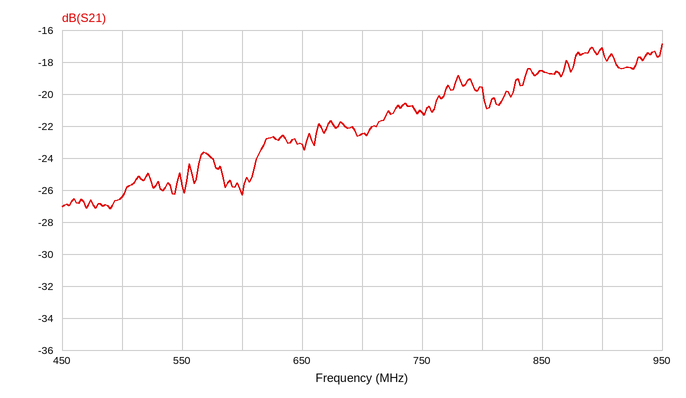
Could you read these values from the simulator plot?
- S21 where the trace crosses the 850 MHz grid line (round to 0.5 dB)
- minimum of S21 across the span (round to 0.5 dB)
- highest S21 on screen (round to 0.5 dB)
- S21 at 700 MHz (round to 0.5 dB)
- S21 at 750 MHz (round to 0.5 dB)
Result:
-18.5 dB
-27.0 dB
-17.0 dB
-22.5 dB
-21.0 dB
